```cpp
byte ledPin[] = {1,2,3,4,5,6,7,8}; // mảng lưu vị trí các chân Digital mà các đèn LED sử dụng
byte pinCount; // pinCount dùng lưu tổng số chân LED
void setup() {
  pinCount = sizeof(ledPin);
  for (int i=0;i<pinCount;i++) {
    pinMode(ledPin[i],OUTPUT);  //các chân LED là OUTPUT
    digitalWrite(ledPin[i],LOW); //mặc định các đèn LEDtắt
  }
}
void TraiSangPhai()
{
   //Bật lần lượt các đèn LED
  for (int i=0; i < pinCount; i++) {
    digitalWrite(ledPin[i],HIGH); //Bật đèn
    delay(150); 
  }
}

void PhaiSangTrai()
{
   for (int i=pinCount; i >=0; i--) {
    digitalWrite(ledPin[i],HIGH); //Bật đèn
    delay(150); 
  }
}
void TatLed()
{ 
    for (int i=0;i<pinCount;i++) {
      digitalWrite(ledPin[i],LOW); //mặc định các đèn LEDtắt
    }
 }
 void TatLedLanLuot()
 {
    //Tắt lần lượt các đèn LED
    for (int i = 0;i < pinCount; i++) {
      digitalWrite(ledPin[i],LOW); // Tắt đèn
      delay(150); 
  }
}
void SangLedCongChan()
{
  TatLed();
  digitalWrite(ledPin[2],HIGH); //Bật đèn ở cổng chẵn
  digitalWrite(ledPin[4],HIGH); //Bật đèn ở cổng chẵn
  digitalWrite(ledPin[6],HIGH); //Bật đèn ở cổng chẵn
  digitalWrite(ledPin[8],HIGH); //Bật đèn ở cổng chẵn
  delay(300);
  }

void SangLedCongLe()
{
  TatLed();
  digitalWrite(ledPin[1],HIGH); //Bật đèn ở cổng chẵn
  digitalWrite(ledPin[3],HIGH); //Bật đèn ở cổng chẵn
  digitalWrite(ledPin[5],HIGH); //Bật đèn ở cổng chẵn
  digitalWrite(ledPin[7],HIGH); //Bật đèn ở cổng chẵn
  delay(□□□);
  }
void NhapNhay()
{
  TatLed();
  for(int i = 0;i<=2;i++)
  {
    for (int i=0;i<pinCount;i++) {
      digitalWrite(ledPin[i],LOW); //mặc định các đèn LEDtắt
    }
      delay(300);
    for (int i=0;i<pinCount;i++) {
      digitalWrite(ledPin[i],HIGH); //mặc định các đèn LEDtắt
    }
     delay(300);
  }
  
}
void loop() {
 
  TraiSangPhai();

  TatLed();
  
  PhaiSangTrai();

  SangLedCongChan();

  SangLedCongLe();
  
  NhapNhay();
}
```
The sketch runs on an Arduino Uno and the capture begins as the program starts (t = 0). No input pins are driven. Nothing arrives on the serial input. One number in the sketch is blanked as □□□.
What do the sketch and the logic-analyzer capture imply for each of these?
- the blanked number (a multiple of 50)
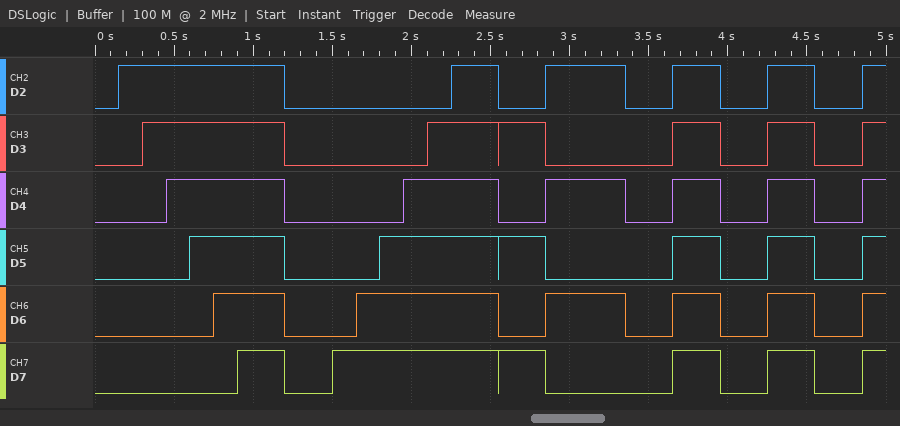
500
